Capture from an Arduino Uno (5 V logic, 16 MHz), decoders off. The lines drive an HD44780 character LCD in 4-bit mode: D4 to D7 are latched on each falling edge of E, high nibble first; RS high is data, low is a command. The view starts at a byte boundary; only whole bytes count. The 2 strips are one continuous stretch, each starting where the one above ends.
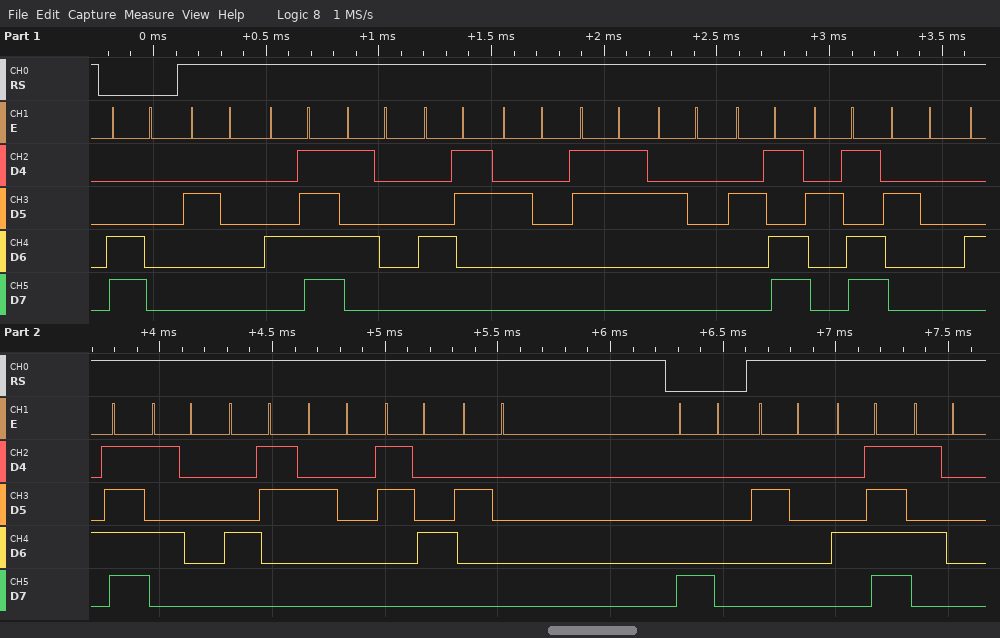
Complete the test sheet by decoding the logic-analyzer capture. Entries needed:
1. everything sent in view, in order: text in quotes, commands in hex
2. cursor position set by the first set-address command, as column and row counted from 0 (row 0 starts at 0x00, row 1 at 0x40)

0xC0 " OPC 3 -- OPC 4 " 0x80 " OP"
column 0, row 1
